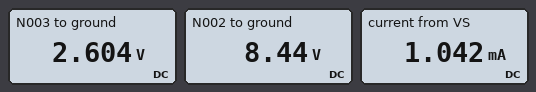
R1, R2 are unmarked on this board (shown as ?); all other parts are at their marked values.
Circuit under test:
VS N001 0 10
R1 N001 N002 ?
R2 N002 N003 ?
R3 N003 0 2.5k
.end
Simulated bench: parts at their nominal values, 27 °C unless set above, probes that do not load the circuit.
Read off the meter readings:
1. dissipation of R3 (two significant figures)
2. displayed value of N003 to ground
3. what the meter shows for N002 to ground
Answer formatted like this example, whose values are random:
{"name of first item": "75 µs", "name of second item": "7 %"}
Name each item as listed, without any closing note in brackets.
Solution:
{"dissipation of R3": "2.7 mW", "displayed value of N003 to ground": "2.604 V", "what the meter shows for N002 to ground": "8.44 V"}
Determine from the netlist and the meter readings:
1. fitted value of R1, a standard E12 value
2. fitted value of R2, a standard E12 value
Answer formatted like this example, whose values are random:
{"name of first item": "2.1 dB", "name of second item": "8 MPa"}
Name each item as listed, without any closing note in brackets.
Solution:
{"fitted value of R1, a standard E12 value": "1.5 kΩ", "fitted value of R2, a standard E12 value": "5.6 kΩ"}
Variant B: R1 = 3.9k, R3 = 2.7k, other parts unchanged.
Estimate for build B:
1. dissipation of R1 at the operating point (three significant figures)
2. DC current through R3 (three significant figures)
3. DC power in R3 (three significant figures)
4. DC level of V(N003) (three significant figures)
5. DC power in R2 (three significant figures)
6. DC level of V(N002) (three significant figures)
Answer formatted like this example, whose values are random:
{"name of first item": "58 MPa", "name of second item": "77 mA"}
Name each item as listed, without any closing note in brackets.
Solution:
{"dissipation of R1 at the operating point": "2.62 mW", "DC current through R3": "820 µA", "DC power in R3": "1.81 mW", "DC level of V(N003)": "2.21 V", "DC power in R2": "3.76 mW", "DC level of V(N002)": "6.80 V"}
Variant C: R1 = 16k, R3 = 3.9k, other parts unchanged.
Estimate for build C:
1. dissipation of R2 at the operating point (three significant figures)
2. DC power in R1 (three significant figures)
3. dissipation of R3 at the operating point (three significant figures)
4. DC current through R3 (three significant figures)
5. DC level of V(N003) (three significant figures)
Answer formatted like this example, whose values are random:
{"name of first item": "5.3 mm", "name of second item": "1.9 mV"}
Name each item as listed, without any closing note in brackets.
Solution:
{"dissipation of R2 at the operating point": "861 µW", "DC power in R1": "2.46 mW", "dissipation of R3 at the operating point": "600 µW", "DC current through R3": "392 µA", "DC level of V(N003)": "1.53 V"}
